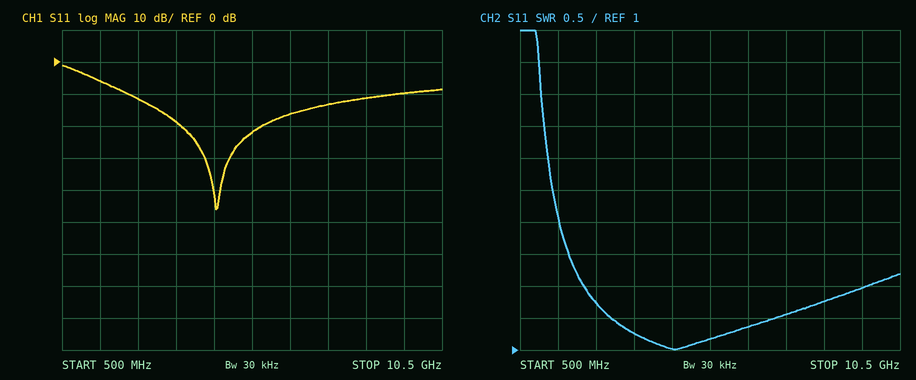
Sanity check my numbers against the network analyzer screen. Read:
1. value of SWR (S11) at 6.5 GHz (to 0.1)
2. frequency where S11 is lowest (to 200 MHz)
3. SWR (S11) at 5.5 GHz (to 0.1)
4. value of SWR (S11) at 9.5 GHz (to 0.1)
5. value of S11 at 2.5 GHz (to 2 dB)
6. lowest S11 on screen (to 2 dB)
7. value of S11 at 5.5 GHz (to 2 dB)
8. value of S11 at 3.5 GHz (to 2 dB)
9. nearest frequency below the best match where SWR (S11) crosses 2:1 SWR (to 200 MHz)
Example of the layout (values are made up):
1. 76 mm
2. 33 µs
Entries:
1. 1.4
2. 4.6 GHz
3. 1.2
4. 2.0
5. -12 dB
6. -46 dB
7. -22 dB
8. -18 dB
9. 2.2 GHz
